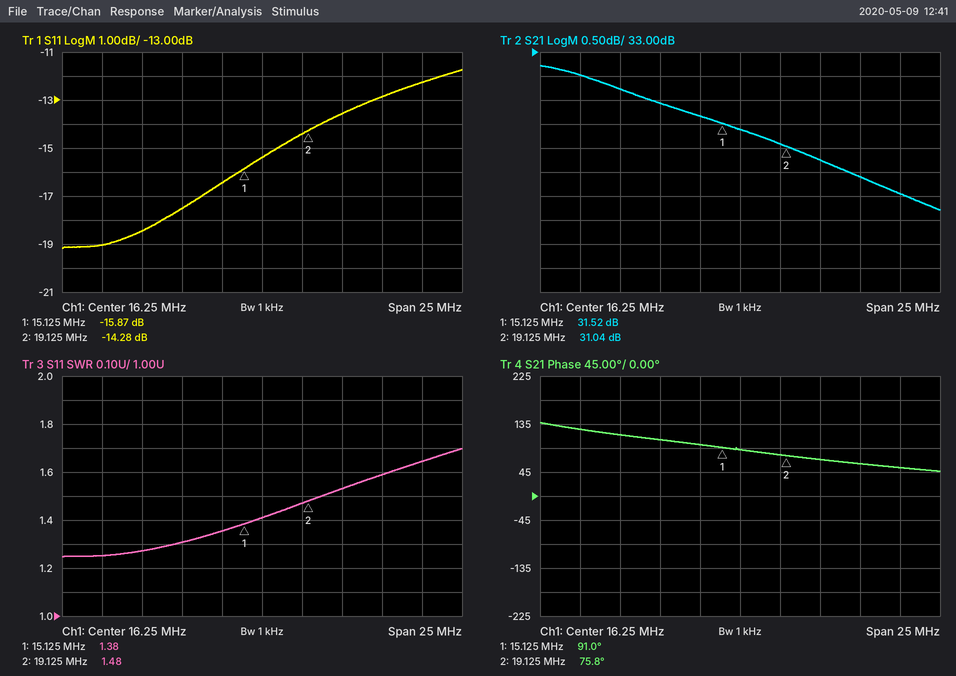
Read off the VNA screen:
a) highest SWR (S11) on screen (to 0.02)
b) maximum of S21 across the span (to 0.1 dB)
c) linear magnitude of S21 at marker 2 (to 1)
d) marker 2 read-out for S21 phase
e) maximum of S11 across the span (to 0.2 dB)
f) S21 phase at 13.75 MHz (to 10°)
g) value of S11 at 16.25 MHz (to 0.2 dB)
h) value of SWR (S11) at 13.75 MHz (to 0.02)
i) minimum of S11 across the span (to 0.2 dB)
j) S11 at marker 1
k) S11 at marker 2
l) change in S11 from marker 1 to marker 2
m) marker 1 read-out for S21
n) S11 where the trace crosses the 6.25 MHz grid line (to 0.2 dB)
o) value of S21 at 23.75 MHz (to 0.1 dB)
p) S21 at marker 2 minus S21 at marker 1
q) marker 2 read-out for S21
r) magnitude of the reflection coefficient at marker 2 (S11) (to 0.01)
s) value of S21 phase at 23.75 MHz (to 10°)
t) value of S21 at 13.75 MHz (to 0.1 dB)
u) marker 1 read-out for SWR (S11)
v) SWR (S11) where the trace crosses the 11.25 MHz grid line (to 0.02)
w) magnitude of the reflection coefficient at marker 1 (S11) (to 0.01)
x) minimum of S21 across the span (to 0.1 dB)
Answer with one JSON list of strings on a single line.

["1.70", "32.7 dB", "36", "75.8°", "-11.8 dB", "100°", "-15.4 dB", "1.36", "-19.2 dB", "-15.87 dB", "-14.28 dB", "1.59 dB", "31.52 dB", "-19.0 dB", "30.4 dB", "-0.48 dB", "31.04 dB", "0.19", "60°", "31.7 dB", "1.38", "1.30", "0.16", "29.7 dB"]
